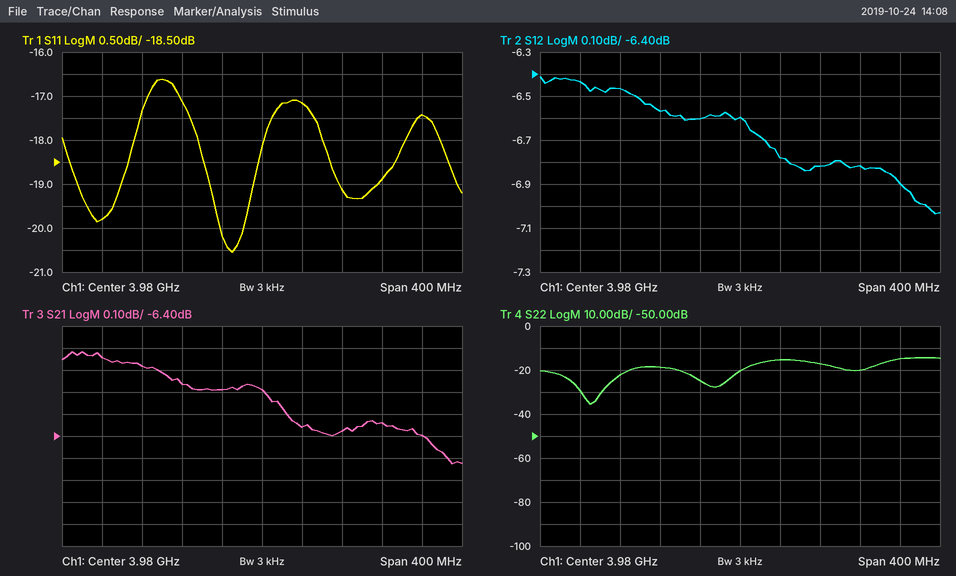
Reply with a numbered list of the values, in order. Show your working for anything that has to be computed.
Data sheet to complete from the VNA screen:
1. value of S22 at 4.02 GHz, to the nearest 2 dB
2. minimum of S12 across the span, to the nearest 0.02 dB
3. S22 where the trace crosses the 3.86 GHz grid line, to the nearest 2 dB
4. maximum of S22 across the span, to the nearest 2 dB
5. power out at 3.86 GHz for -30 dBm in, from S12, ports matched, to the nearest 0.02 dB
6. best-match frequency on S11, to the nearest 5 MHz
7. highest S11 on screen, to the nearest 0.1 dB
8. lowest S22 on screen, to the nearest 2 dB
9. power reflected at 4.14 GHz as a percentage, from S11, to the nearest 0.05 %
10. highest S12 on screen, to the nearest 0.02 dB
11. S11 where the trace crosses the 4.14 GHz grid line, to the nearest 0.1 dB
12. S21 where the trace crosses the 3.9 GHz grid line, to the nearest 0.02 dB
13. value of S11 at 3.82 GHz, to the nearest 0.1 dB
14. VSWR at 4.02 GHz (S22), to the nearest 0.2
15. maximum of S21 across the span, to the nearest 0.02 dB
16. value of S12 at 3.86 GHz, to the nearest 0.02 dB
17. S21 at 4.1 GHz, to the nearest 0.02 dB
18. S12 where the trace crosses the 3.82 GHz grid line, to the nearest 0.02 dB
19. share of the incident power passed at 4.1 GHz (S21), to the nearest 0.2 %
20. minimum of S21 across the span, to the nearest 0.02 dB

1. -16 dB
2. -7.04 dB
3. -22 dB
4. -14 dB
5. -30 dBm + (-6.46 dB) = -36.46 dBm
6. 3.950 GHz
7. -16.6 dB
8. -36 dB
9. 10^(-17.4/10) ≈ 1.82 %, so 1.80 % to the nearest 0.05 %
10. -6.42 dB
11. -17.4 dB
12. -6.16 dB
13. -19.8 dB
14. |Γ| = 10^(-16/20) = 0.1585; VSWR = (1 + 0.1585)/(1 − 0.1585) ≈ 1.4
15. -6.02 dB
16. -6.46 dB
17. -6.34 dB
18. -6.44 dB
19. 10^(-6.34/10) ≈ 23.2 %
20. -6.52 dB
